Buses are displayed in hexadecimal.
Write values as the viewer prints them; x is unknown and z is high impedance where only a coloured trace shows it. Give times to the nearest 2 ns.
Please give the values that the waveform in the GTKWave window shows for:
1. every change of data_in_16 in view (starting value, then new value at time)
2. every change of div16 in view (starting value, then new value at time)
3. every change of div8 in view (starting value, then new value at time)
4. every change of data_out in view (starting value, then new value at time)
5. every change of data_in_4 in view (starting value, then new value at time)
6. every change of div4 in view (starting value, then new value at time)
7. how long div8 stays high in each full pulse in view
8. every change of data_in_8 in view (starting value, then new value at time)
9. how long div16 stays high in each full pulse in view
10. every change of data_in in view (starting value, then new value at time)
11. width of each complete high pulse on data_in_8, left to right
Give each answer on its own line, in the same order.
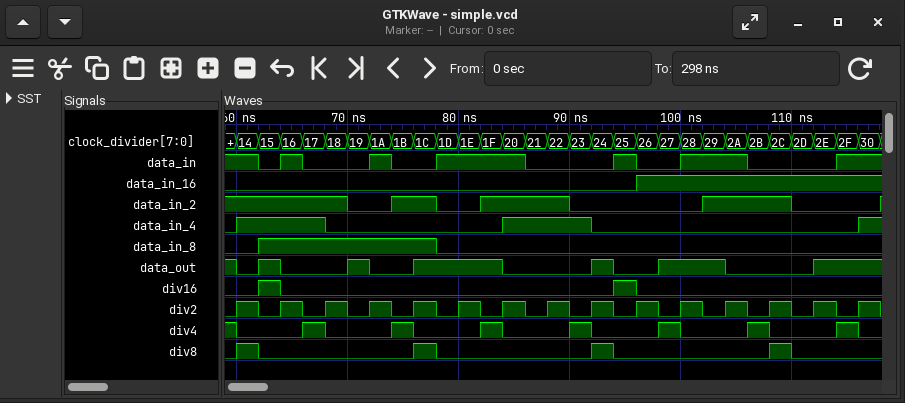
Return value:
0, 1 at 96 ns
0, 1 at 62 ns, 0 at 64 ns, 1 at 94 ns, 0 at 96 ns
0, 1 at 60 ns, 0 at 62 ns, 1 at 76 ns, 0 at 78 ns, 1 at 92 ns, 0 at 94 ns, 1 at 108 ns, 0 at 110 ns
1, 0 at 60 ns, 1 at 62 ns, 0 at 64 ns, 1 at 70 ns, 0 at 72 ns, 1 at 76 ns, 0 at 84 ns, 1 at 92 ns, 0 at 94 ns, 1 at 98 ns, 0 at 104 ns, 1 at 112 ns
0, 1 at 60 ns, 0 at 68 ns, 1 at 84 ns, 0 at 92 ns, 1 at 116 ns
1, 0 at 60 ns, 1 at 66 ns, 0 at 68 ns, 1 at 74 ns, 0 at 76 ns, 1 at 82 ns, 0 at 84 ns, 1 at 90 ns, 0 at 92 ns, 1 at 98 ns, 0 at 100 ns, 1 at 106 ns, 0 at 108 ns, 1 at 114 ns, 0 at 116 ns
2 ns, 2 ns, 2 ns, 2 ns
0, 1 at 62 ns, 0 at 78 ns
2 ns, 2 ns
1, 0 at 62 ns, 1 at 64 ns, 0 at 66 ns, 1 at 72 ns, 0 at 74 ns, 1 at 78 ns, 0 at 86 ns, 1 at 94 ns, 0 at 96 ns, 1 at 100 ns, 0 at 106 ns, 1 at 114 ns
16 ns
